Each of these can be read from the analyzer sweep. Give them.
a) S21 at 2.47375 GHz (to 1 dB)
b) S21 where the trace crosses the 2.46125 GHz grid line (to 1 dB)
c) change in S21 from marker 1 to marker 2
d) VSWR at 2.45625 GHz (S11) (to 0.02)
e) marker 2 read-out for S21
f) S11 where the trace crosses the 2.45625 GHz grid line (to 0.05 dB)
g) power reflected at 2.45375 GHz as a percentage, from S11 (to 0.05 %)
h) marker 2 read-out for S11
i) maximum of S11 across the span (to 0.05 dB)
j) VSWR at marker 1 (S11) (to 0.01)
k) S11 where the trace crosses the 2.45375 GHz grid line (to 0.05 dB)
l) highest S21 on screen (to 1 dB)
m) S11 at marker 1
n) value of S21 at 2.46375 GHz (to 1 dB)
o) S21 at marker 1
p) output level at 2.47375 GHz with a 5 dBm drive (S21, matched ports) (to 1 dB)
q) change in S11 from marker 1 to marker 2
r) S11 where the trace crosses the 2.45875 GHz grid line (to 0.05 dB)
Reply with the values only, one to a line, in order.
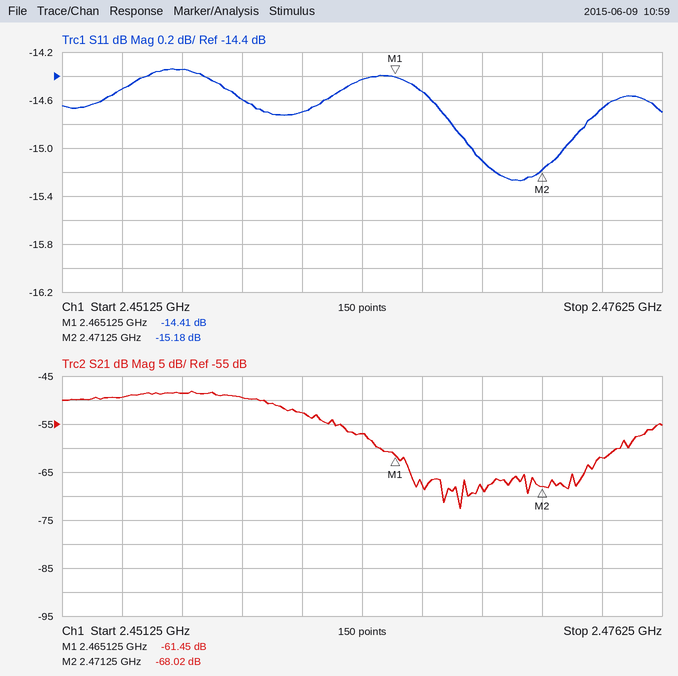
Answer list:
-62 dB
-53 dB
-6.57 dB
1.48
-68.02 dB
-14.35 dB
3.55 %
-15.18 dB
-14.35 dB
1.47
-14.50 dB
-48 dB
-14.41 dB
-57 dB
-61.45 dB
-57 dBm
-0.77 dB
-14.60 dB
